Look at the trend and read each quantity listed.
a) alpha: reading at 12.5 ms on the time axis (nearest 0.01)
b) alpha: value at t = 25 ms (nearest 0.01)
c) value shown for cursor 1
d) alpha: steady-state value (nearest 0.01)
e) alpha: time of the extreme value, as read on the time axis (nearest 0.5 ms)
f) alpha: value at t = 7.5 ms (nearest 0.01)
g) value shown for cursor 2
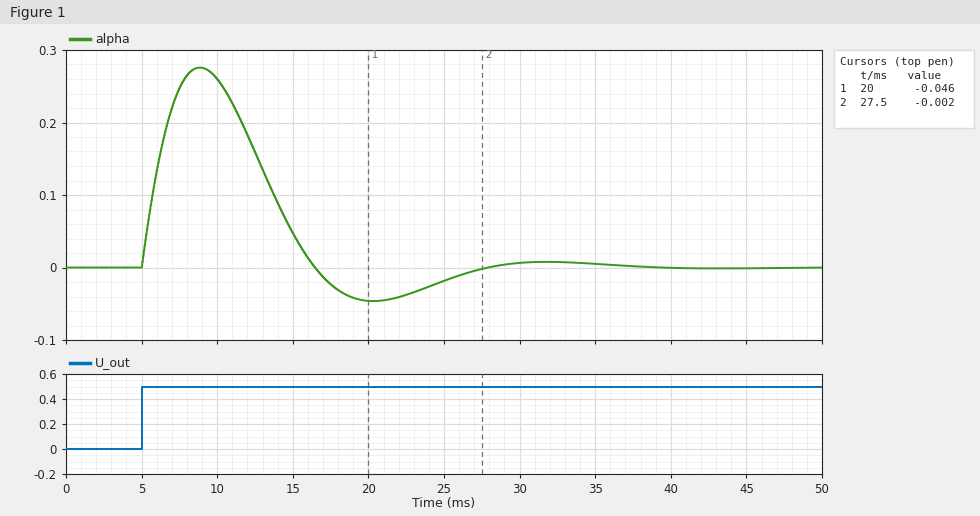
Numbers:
0.16
-0.02
-0.046
0.00
9.0 ms
0.25
-0.002
